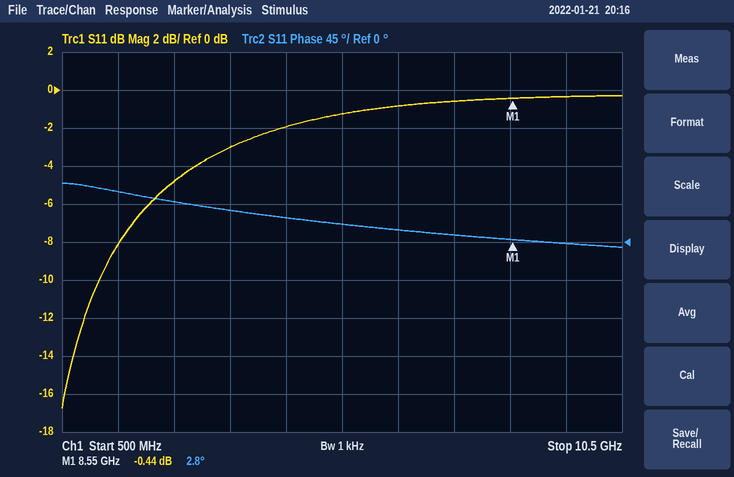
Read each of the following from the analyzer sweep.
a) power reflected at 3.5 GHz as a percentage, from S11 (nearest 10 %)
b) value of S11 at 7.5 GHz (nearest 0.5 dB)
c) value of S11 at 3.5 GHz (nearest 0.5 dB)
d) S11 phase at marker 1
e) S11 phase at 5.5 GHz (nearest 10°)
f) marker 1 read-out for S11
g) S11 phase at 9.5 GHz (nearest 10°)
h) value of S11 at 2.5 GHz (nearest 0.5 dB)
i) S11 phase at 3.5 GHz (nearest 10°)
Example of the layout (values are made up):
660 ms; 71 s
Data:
50 %; -0.5 dB; -3.0 dB; 2.8°; 20°; -0.44 dB; 0°; -5.0 dB; 40°
